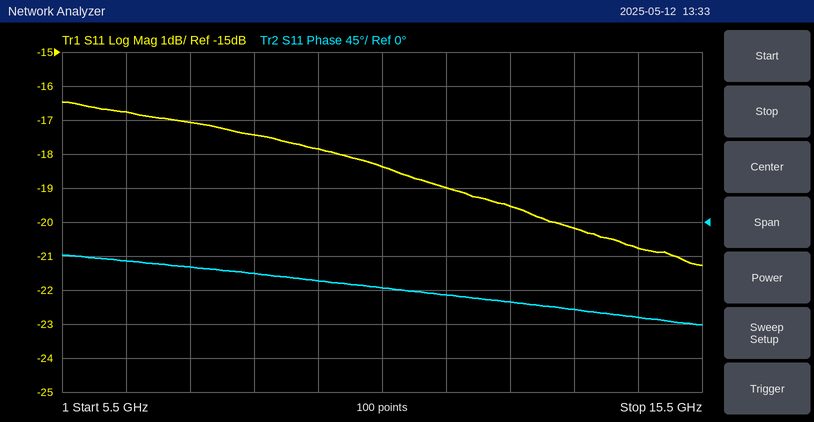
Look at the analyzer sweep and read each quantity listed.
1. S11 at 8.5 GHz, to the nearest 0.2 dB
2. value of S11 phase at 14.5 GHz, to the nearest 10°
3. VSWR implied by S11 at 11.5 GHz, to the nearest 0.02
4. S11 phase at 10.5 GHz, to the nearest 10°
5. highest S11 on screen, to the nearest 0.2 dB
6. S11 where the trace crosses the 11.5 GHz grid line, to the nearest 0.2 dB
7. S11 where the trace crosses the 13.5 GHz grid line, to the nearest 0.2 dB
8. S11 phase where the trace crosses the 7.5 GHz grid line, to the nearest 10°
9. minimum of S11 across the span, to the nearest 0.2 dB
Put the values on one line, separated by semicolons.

-17.4 dB; -130°; 1.26; -90°; -16.4 dB; -19.0 dB; -20.2 dB; -60°; -21.2 dB
